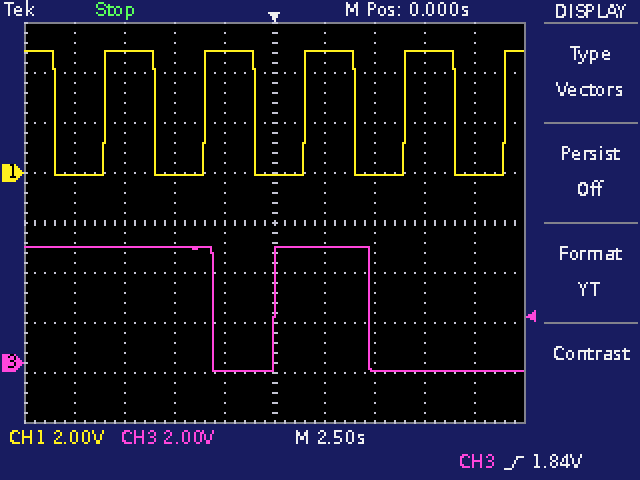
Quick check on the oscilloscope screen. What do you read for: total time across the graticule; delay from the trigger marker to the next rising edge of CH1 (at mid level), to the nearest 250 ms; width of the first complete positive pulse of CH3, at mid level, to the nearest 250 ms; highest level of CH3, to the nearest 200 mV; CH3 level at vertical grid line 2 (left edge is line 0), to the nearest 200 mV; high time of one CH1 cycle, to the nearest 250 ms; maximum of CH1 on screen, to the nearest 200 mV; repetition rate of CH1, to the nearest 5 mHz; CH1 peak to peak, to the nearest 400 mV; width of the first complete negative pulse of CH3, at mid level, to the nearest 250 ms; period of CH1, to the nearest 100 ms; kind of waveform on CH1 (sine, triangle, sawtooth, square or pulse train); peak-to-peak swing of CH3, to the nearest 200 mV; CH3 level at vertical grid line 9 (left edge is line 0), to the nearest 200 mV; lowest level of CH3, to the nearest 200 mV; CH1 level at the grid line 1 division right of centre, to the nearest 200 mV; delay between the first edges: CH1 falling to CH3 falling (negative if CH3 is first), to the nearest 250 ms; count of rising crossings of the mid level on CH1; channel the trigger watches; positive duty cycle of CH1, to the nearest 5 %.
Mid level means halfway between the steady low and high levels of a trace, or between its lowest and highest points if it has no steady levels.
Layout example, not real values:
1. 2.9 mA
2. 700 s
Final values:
1. 25 s
2. 1.50 s
3. 4.75 s
4. 4.6 V
5. 4.6 V
6. 2.50 s
7. 4.8 V
8. 200 mHz
9. 4.8 V
10. 3.00 s
11. 5.0 s
12. square
13. 5.0 V
14. -400 mV
15. -400 mV
16. 4.8 V
17. +8.00 s
18. 5
19. CH3
20. 50 %
